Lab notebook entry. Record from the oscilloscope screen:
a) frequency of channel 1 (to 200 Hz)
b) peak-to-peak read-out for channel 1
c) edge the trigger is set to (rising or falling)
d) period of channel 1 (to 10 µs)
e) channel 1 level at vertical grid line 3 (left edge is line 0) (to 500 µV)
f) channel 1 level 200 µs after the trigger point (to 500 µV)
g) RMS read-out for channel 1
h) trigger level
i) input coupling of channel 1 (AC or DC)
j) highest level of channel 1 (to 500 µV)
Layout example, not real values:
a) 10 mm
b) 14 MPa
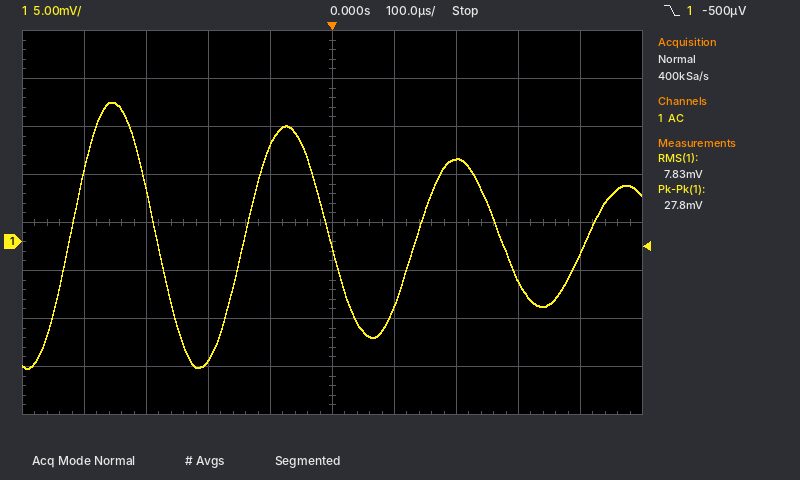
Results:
a) 3.6 kHz
b) 27.8 mV
c) falling
d) 280 µs
e) -12.5 mV
f) 8.5 mV
g) 7.83 mV
h) -500 µV
i) AC
j) 14.5 mV
